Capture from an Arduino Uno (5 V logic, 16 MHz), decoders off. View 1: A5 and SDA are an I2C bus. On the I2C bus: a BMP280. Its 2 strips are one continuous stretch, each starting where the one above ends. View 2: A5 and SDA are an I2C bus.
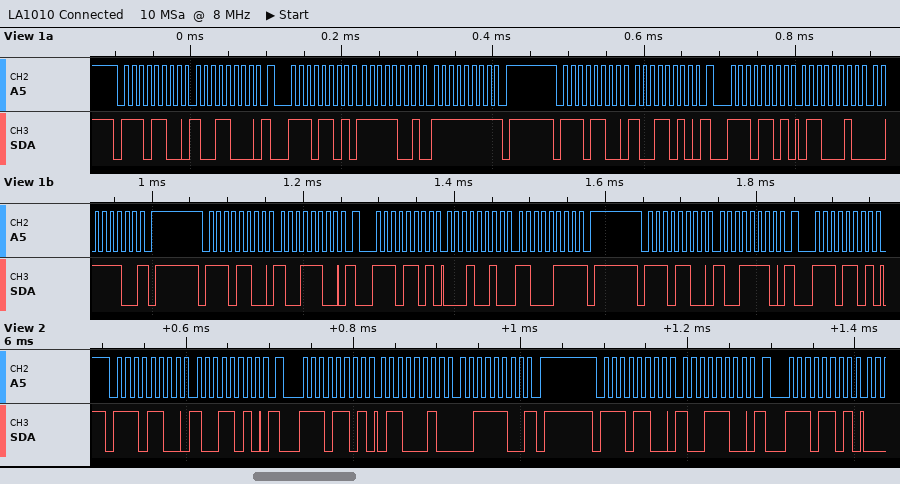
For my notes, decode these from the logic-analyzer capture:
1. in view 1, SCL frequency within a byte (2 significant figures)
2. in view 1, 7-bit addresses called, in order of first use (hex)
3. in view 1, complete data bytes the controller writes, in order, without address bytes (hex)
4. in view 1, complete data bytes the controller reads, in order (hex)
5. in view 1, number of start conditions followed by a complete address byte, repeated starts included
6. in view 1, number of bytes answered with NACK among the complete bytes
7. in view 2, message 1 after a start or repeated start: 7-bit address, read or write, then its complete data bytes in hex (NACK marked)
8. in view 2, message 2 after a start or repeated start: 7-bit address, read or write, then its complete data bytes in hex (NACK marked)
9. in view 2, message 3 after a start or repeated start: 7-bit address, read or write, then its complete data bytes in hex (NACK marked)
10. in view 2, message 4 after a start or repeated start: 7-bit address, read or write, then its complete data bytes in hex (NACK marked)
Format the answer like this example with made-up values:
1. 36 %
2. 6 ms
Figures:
1. 100 kHz
2. 0x76
3. 98 9A 9C 9E
4. F9 FF 62 3C 12 C7
5. 8
6. 3
7. 0x76 write: 9A
8. 0x76 read: 62 3C NACK
9. 0x76 write: 9C
10. 0x76 read
